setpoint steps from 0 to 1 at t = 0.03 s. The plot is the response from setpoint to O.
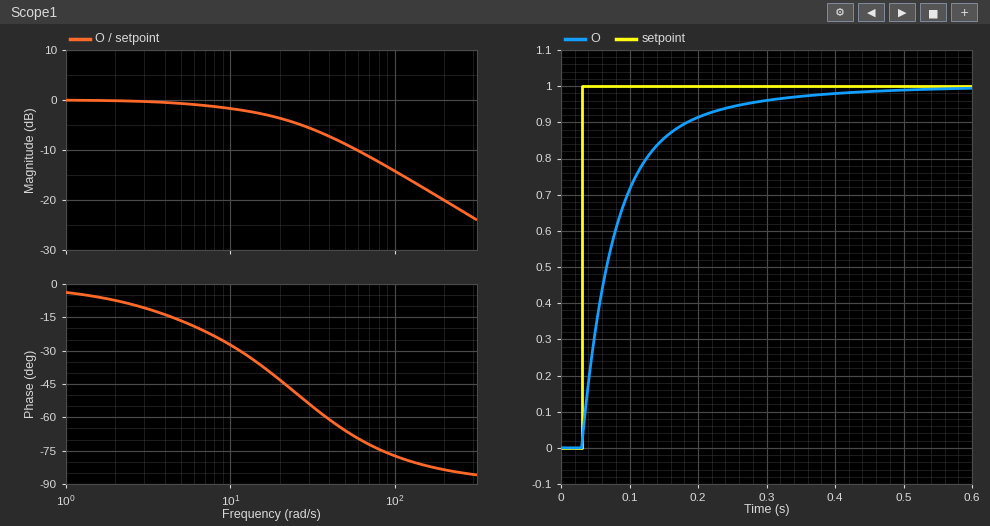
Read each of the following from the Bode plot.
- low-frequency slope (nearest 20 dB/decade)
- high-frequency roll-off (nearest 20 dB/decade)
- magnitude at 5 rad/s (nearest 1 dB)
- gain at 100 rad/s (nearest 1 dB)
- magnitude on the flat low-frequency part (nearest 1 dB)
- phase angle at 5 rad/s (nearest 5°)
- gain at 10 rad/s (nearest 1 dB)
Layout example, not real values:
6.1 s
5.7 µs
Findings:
0 dB/decade
-20 dB/decade
-1 dB
-14 dB
0 dB
-15°
-2 dB
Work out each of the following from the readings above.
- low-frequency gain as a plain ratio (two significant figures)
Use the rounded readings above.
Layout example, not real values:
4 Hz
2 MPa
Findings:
1.0
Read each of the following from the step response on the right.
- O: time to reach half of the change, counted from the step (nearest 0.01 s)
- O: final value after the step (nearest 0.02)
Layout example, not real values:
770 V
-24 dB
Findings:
0.04 s
1.00
